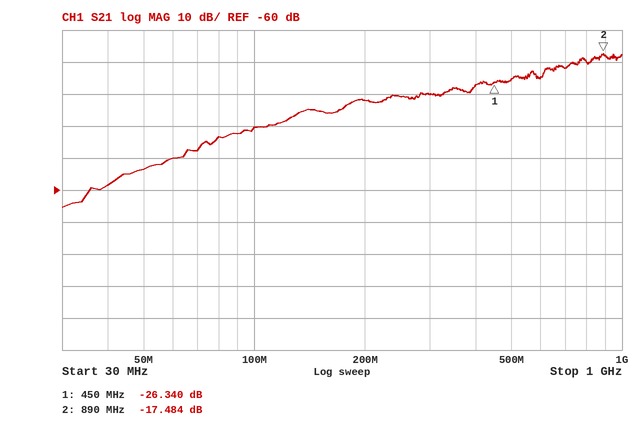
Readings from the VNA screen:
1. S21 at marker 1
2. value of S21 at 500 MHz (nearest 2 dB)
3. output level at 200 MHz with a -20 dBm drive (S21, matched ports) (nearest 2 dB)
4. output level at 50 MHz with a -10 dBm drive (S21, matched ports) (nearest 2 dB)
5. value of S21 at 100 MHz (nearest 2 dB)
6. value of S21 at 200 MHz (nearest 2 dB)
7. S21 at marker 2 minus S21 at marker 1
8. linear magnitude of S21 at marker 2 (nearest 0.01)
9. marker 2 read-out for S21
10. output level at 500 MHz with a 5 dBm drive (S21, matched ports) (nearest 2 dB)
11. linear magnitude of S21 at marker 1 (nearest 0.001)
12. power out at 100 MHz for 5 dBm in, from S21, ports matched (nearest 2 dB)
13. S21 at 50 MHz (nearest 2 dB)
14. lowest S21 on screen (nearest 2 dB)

-26.340 dB
-26 dB
-52 dBm
-64 dBm
-40 dB
-32 dB
8.856 dB
0.13
-17.484 dB
-20 dBm
0.048
-36 dBm
-54 dB
-66 dB
